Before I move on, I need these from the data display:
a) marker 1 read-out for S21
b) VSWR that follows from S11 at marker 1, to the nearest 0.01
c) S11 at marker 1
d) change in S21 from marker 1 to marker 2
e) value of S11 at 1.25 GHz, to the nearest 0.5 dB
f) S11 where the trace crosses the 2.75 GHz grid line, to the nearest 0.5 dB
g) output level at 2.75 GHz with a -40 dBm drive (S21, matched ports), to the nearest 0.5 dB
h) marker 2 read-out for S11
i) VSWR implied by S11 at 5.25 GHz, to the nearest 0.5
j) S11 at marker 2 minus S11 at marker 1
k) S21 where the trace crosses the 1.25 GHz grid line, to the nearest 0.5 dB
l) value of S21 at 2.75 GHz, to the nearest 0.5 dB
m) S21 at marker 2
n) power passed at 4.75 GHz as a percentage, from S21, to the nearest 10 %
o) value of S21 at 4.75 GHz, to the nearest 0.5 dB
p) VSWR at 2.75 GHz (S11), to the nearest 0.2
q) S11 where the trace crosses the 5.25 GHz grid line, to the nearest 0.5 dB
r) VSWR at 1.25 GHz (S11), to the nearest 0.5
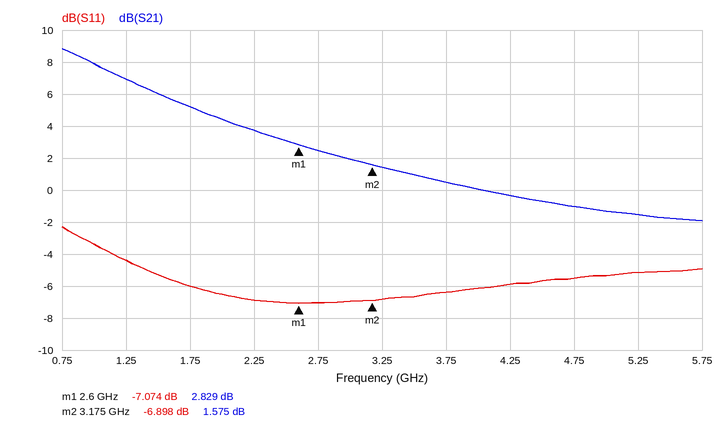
2.829 dB
2.59
-7.074 dB
-1.254 dB
-4.5 dB
-7.0 dB
-37.5 dBm
-6.898 dB
3.5
0.176 dB
7.0 dB
2.5 dB
1.575 dB
80 %
-1.0 dB
2.6
-5.0 dB
4.0
